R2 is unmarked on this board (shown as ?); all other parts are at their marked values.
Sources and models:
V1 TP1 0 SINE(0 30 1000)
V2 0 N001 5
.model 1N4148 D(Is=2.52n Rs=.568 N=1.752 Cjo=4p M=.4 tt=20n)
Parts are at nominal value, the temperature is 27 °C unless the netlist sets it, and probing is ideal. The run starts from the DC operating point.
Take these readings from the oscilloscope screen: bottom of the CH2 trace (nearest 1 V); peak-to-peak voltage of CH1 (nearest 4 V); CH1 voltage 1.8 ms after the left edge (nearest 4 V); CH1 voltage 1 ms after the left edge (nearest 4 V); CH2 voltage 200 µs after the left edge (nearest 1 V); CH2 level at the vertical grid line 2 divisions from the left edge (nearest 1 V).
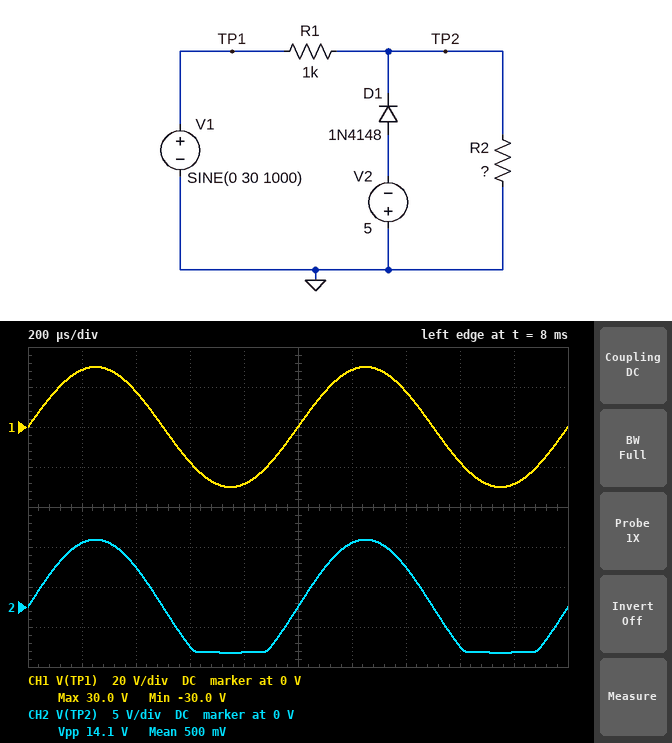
-6 V
60 V
-28 V
0 V
8 V
5 V
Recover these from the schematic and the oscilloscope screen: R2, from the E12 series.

390 Ω
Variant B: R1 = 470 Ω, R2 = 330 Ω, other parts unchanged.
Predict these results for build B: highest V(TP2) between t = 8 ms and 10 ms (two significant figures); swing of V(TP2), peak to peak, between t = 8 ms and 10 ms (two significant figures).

12 V
18 V
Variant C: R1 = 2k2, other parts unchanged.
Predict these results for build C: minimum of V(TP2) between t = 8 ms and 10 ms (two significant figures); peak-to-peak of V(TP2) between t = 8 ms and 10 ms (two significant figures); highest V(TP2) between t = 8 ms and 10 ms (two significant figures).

-4.5 V
9.0 V
4.5 V
